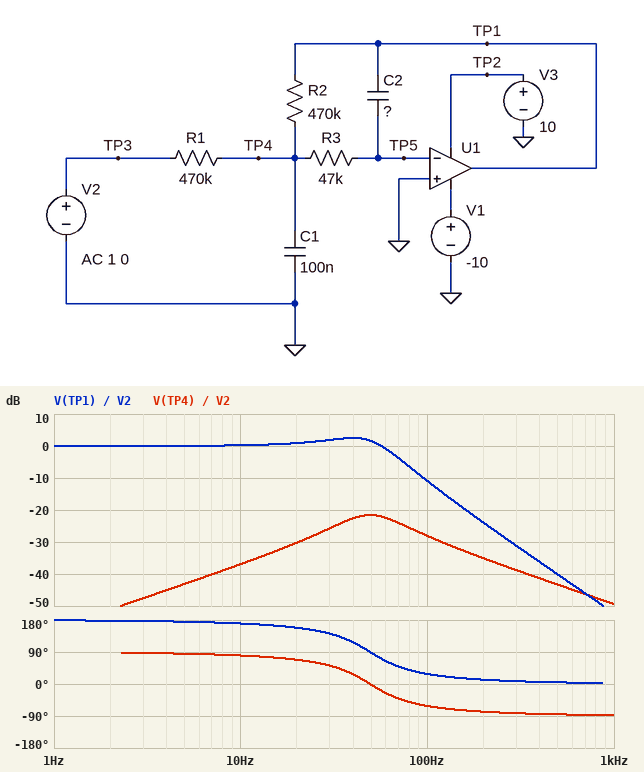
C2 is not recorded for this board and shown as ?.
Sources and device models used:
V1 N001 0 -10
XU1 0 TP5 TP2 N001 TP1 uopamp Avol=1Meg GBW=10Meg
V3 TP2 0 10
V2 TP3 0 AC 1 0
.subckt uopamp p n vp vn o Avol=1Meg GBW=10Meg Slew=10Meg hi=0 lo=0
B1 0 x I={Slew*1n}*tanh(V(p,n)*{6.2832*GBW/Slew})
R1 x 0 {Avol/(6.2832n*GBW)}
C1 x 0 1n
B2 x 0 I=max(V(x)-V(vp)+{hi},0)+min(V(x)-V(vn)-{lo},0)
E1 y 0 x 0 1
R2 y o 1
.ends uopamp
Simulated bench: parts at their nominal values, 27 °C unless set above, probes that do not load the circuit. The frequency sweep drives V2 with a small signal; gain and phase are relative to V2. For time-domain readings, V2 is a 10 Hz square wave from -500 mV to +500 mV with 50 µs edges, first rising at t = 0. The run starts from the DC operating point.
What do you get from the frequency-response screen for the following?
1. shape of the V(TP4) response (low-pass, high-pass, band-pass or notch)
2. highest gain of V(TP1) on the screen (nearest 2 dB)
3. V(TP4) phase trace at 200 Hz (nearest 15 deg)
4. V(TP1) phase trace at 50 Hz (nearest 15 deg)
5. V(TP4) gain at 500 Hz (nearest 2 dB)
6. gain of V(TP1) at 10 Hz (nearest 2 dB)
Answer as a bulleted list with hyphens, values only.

- band-pass
- 2 dB
- -75 deg
- 90 deg
- -44 dB
- 0 dB
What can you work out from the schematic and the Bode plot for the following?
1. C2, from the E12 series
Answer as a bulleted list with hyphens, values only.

- 4.7 nF
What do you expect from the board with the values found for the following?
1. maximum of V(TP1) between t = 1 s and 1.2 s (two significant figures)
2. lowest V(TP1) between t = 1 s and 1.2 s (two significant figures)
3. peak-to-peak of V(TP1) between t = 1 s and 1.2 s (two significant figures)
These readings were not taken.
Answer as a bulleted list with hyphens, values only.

- 740 mV
- -740 mV
- 1.5 V
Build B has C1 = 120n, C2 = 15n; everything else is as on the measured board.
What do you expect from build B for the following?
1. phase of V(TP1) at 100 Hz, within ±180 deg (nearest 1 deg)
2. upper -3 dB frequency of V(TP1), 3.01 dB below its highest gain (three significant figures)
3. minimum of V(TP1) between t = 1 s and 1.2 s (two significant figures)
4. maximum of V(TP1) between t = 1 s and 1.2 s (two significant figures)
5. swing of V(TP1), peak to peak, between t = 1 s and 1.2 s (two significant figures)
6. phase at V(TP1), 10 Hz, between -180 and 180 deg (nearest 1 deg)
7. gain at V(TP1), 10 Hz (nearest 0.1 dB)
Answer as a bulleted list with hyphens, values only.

- 20 deg
- 26.4 Hz
- -560 mV
- 560 mV
- 1.1 V
- 148 deg
- 0 dB
